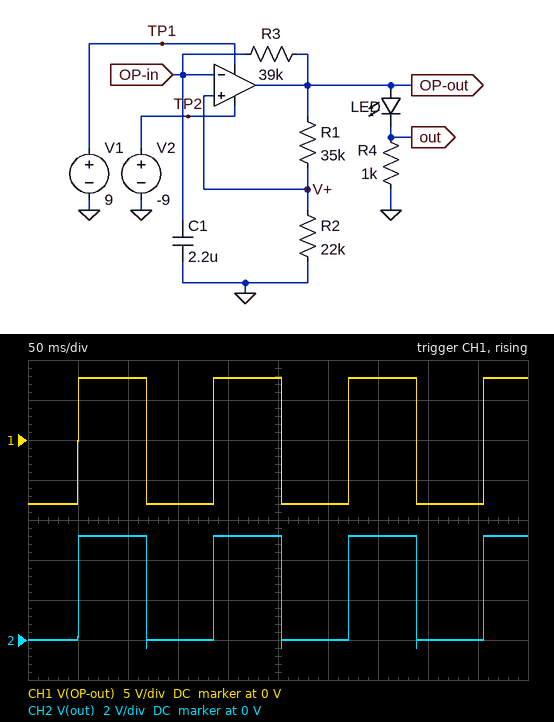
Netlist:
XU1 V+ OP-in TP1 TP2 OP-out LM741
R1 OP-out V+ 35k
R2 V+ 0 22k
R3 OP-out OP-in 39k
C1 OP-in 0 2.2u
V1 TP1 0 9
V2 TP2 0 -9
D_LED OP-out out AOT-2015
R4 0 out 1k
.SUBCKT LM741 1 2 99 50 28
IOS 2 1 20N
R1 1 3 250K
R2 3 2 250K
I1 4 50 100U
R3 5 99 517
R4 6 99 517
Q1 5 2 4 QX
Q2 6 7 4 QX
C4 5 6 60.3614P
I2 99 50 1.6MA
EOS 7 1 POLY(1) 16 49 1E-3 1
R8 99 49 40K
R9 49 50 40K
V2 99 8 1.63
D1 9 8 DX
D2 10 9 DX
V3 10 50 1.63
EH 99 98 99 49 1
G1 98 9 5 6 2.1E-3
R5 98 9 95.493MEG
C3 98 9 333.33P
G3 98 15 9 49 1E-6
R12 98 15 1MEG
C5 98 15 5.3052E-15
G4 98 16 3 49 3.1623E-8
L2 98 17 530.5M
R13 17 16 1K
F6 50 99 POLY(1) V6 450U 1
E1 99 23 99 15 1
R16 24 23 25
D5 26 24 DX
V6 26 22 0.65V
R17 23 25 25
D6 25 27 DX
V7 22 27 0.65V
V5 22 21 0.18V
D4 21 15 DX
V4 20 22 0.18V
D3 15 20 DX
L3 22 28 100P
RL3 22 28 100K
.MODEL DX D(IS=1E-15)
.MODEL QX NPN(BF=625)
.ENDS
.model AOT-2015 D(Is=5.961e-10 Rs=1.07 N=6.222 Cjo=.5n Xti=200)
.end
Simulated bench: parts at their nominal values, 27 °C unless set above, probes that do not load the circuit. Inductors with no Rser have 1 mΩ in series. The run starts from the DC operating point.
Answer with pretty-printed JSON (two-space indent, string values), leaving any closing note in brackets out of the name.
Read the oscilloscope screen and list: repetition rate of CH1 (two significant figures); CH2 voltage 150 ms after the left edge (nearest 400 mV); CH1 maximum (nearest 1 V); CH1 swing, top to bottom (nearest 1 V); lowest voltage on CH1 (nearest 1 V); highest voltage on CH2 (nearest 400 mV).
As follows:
{
  "repetition rate of CH1": "7.4 Hz",
  "CH2 voltage 150 ms after the left edge": "0 V",
  "CH1 maximum": "8 V",
  "CH1 swing, top to bottom": "16 V",
  "lowest voltage on CH1": "-8 V",
  "highest voltage on CH2": "5.2 V"
}
